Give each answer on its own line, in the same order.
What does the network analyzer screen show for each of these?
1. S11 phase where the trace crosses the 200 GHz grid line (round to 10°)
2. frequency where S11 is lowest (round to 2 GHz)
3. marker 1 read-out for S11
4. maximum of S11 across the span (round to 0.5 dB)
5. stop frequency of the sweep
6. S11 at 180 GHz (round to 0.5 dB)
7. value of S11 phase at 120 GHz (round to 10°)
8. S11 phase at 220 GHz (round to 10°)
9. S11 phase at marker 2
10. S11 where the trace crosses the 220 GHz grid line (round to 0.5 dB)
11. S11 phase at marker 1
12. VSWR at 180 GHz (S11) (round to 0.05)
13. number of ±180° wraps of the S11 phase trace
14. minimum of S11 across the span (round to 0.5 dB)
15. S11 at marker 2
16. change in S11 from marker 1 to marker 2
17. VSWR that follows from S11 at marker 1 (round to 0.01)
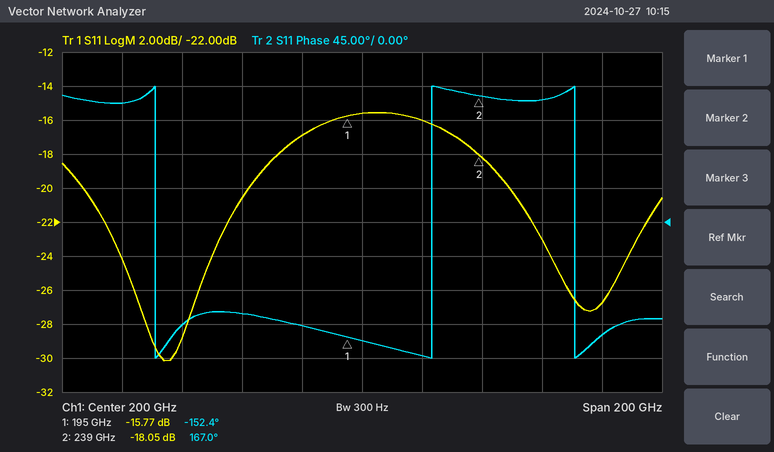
-160°
134 GHz
-15.77 dB
-15.5 dB
300 GHz
-17.0 dB
160°
-180°
167.0°
-16.0 dB
-152.4°
1.35
3
-30.0 dB
-18.05 dB
-2.28 dB
1.39
